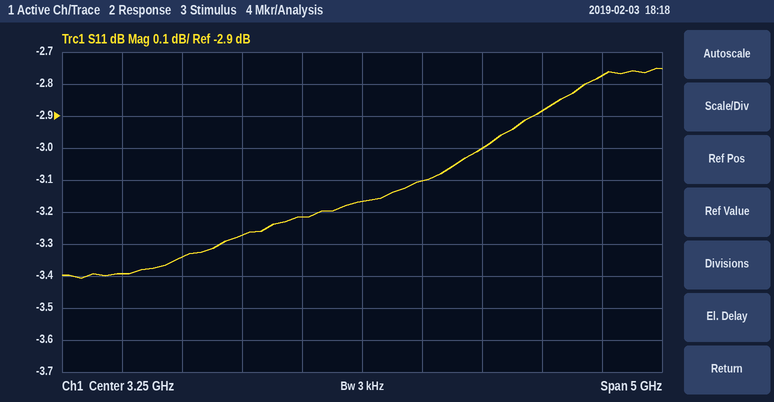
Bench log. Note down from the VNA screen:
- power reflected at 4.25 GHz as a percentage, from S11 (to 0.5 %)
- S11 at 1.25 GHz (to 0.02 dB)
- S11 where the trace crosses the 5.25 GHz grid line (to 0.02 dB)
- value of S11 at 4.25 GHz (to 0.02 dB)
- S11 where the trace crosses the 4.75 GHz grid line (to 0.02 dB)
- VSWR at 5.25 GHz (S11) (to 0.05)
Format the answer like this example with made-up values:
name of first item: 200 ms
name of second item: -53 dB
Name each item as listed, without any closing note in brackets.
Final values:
power reflected at 4.25 GHz as a percentage, from S11: 50.0 %
S11 at 1.25 GHz: -3.40 dB
S11 where the trace crosses the 5.25 GHz grid line: -2.78 dB
value of S11 at 4.25 GHz: -3.00 dB
S11 where the trace crosses the 4.75 GHz grid line: -2.88 dB
VSWR at 5.25 GHz (S11): 6.30
